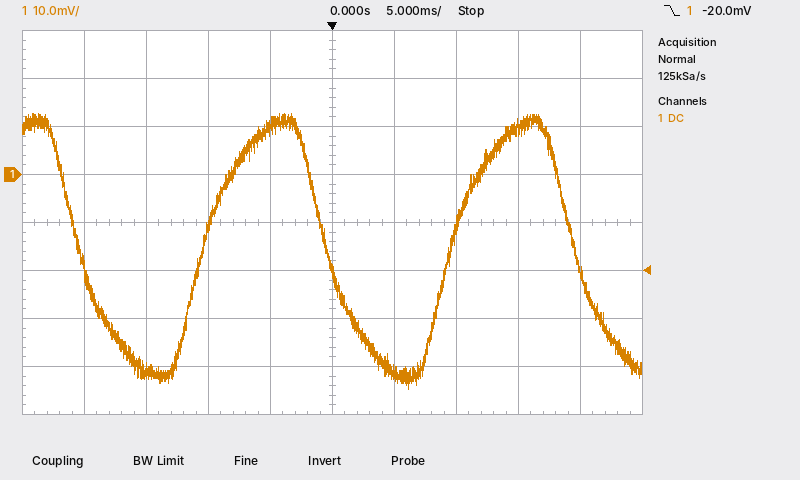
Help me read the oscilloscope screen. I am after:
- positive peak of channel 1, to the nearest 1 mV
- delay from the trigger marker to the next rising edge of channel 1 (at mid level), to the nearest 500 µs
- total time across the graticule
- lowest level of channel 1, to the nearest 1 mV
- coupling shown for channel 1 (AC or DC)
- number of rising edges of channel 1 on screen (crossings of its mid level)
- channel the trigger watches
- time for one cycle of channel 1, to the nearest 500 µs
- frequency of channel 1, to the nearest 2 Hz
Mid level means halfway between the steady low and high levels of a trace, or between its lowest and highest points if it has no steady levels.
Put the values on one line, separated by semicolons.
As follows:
13 mV; 9.5 ms; 50 ms; -45 mV; DC; 2; channel 1; 20.0 ms; 50 Hz
